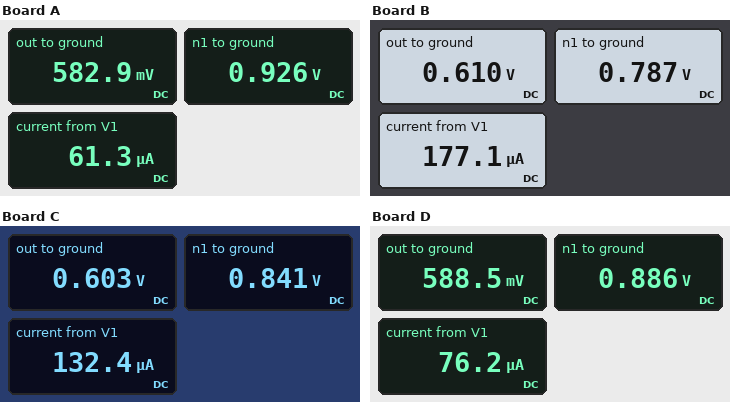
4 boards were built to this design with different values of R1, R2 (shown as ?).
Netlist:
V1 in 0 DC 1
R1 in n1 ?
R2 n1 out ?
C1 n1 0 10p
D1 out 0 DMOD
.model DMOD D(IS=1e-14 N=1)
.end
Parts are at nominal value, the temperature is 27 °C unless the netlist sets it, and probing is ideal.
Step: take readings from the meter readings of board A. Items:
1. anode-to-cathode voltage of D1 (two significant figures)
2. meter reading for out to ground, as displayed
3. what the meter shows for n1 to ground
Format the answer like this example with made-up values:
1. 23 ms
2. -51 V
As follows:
1. 580 mV
2. 582.9 mV
3. 0.926 V
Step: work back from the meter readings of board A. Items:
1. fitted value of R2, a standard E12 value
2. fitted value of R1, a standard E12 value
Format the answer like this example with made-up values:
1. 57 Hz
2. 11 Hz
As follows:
1. 5.6 kΩ
2. 1.2 kΩ
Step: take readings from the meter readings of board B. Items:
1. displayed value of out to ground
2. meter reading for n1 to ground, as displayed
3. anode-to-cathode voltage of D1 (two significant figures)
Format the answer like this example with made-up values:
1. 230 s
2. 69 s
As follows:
1. 0.610 V
2. 0.787 V
3. 610 mV
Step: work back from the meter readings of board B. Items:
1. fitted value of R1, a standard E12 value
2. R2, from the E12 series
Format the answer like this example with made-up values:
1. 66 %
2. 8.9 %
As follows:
1. 1.2 kΩ
2. 1 kΩ
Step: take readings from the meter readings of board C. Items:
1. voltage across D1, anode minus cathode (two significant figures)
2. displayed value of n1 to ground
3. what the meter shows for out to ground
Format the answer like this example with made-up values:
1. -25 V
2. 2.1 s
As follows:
1. 600 mV
2. 0.841 V
3. 0.603 V
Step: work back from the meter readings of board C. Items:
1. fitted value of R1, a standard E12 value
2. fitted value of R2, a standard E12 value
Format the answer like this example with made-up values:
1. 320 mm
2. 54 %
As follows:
1. 1.2 kΩ
2. 1.8 kΩ
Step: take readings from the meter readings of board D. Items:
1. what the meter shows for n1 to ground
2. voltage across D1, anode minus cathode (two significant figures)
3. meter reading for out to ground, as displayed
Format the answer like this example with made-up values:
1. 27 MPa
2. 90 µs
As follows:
1. 0.886 V
2. 590 mV
3. 588.5 mV
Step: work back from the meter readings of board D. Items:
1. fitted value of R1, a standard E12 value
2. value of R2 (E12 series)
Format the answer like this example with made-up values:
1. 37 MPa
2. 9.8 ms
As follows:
1. 1.5 kΩ
2. 3.9 kΩ
